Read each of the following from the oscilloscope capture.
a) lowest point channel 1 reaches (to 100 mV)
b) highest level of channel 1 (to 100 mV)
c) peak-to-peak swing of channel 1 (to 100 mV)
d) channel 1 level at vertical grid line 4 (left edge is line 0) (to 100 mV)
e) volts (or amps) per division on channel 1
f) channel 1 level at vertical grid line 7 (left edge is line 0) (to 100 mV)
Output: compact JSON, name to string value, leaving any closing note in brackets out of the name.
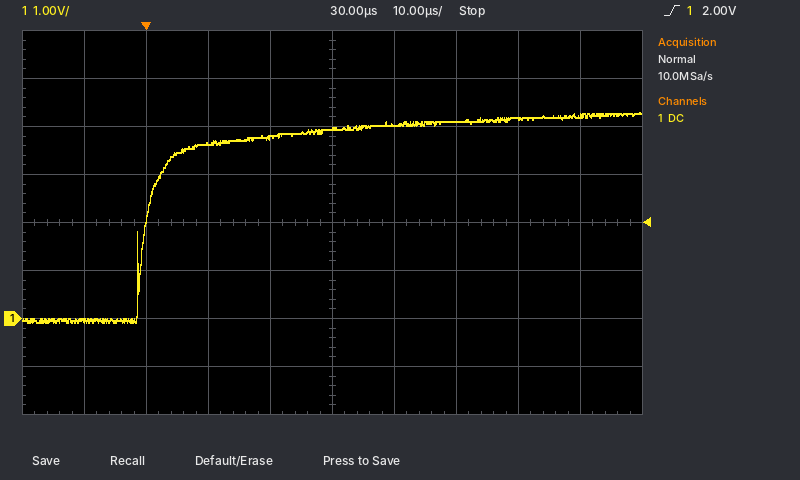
{"lowest point channel 1 reaches": "-100 mV", "highest level of channel 1": "4.3 V", "peak-to-peak swing of channel 1": "4.4 V", "channel 1 level at vertical grid line 4 (left edge is line 0)": "3.8 V", "volts (or amps) per division on channel 1": "1 V", "channel 1 level at vertical grid line 7 (left edge is line 0)": "4.1 V"}
